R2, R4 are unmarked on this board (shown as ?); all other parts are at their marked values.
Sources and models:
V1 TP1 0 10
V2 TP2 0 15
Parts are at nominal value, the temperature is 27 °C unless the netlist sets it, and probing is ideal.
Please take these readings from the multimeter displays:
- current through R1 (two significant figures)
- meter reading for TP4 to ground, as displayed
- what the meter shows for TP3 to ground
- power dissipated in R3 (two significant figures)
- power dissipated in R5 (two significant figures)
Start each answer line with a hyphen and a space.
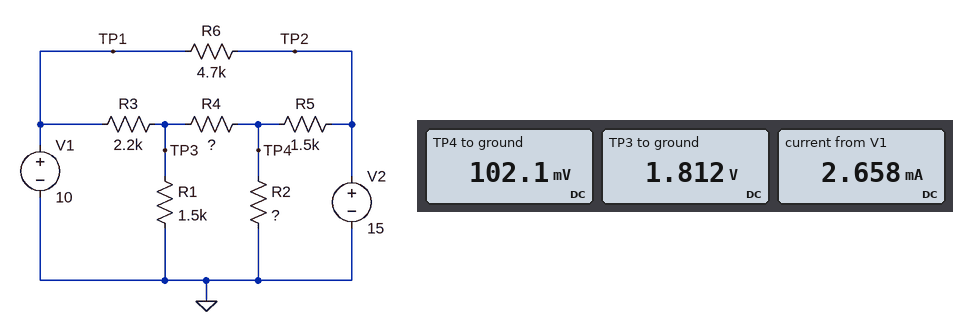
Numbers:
- 1.2 mA
- 102.1 mV
- 1.812 V
- 30 mW
- 150 mW
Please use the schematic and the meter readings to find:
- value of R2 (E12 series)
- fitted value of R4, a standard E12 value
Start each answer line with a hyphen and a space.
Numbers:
- 8.2 Ω
- 680 Ω
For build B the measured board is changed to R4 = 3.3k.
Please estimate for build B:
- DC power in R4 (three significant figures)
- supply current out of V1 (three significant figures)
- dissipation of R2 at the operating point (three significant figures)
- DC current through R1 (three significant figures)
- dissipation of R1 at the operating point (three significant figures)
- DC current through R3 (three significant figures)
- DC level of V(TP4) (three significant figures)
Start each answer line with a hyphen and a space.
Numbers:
- 2.95 mW
- 2.02 mA
- 972 µW
- 2.14 mA
- 6.87 mW
- 3.09 mA
- 89.3 mV
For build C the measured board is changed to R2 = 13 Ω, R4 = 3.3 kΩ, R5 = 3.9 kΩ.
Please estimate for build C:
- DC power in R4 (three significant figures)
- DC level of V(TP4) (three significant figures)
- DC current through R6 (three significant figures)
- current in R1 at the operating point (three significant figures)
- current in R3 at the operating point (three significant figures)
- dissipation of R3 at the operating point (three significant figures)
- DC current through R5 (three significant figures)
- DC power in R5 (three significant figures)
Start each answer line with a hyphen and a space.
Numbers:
- 2.99 mW
- 62.2 mV
- 1.06 mA
- 2.14 mA
- 3.09 mA
- 21.0 mW
- 3.83 mA
- 57.2 mW
